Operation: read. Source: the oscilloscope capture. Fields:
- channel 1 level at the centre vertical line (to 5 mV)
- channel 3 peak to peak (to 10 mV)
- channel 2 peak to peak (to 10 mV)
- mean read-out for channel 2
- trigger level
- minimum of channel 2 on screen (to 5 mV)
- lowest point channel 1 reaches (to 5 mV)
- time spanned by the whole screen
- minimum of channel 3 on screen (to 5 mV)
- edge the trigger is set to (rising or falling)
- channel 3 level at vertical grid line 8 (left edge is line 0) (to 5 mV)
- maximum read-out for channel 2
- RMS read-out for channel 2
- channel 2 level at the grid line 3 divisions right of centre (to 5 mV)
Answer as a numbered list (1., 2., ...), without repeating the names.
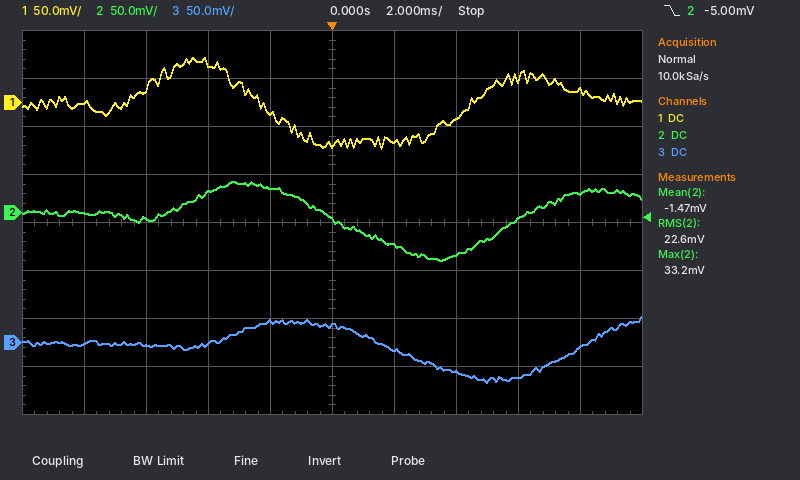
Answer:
1. -45 mV
2. 70 mV
3. 80 mV
4. -1.47 mV
5. -5.00 mV
6. -50 mV
7. -50 mV
8. 20 ms
9. -40 mV
10. falling
11. -35 mV
12. 33.2 mV
13. 22.6 mV
14. -5 mV
